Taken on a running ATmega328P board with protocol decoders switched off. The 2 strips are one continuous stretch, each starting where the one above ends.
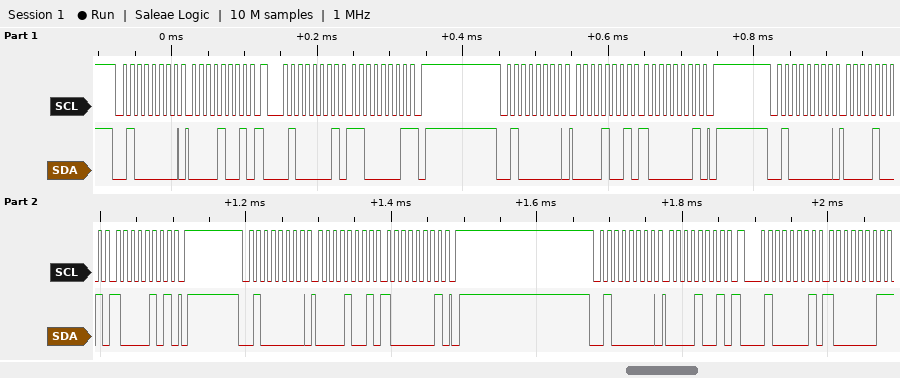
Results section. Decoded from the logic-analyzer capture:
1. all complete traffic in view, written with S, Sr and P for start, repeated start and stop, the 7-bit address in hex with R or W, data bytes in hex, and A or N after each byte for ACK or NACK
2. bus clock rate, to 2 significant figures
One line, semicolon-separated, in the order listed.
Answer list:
S 20W A 09 A Sr 20R A C1 N P S 20W A 09 A 81 A P S 20W A 09 A 85 A P S 20W A 09 A 81 A P S 20W A 09 A Sr 20R A 81 N; 100 kHz
